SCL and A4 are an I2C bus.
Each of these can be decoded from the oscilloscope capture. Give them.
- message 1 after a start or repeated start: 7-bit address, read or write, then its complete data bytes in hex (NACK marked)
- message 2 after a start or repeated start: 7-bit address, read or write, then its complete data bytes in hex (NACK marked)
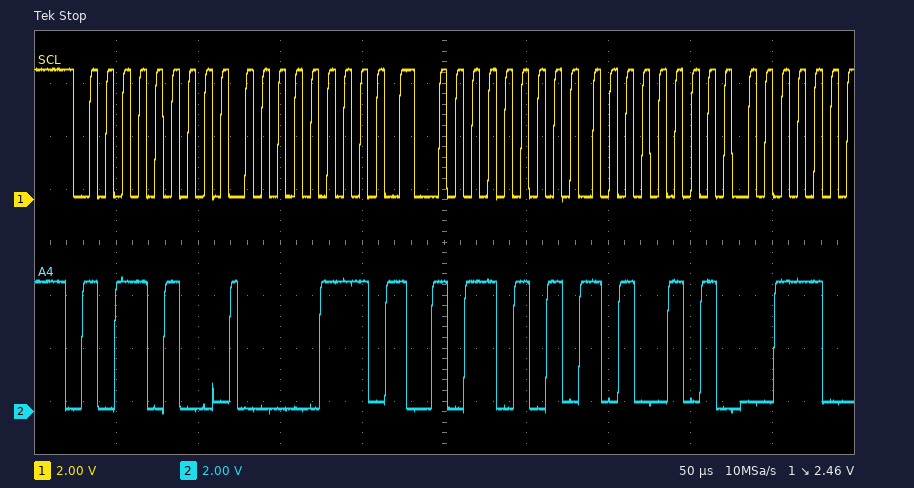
0x5A write: 07
0x5A read: A5
